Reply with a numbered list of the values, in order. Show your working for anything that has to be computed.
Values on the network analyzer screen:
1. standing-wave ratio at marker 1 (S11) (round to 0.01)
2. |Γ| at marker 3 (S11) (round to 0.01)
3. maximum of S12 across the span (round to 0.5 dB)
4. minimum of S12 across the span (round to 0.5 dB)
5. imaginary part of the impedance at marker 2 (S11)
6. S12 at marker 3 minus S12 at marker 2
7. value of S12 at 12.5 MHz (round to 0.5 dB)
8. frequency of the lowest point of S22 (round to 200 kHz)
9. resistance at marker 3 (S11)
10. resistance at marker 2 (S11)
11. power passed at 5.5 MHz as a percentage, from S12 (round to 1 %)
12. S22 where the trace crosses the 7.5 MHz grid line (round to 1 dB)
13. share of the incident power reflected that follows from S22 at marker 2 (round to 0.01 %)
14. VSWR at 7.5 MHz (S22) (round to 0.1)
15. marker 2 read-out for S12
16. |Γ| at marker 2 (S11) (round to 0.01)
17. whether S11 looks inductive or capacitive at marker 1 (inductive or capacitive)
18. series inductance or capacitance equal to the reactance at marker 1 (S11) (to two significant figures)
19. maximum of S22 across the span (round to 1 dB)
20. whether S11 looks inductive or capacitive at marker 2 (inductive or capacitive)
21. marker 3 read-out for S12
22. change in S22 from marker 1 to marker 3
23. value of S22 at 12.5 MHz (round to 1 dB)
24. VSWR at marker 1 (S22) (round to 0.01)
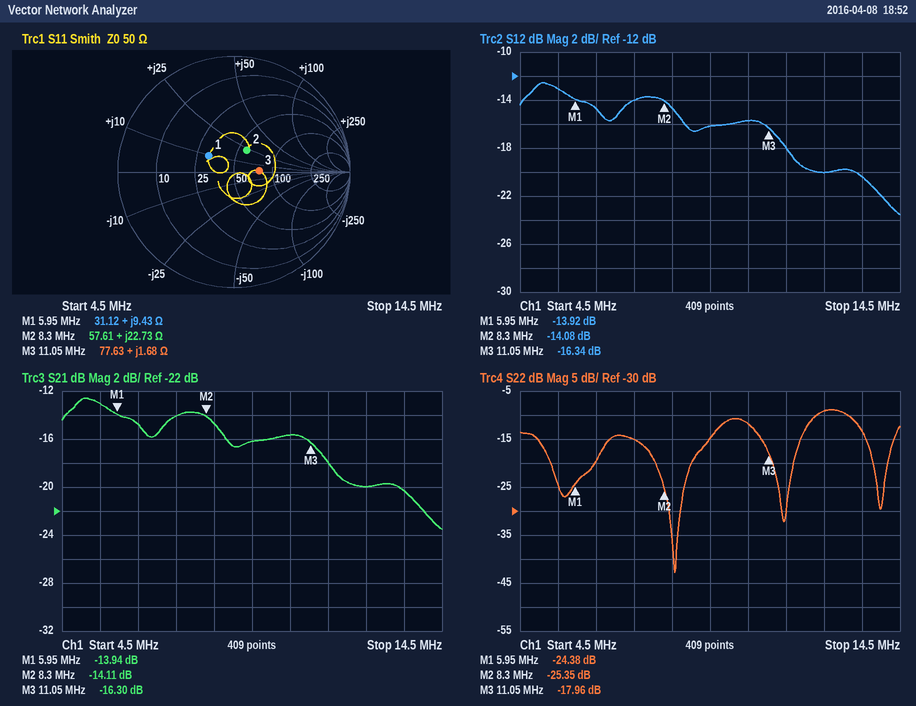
1. 1.70
2. 0.22
3. -12.5 dB
4. -23.5 dB
5. +22.73 Ω
6. -16.34 − (-14.08) = -2.26 dB
7. -20.0 dB
8. 8.6 MHz
9. 77.63 Ω
10. 57.61 Ω
11. 10^(-13/10) ≈ 5 %
12. -15 dB
13. 10^(-25.35/10) ≈ 0.29 %
14. |Γ| = 10^(-15/20) = 0.1778; VSWR = (1 + 0.1778)/(1 − 0.1778) ≈ 1.4
15. -14.08 dB
16. 0.22
17. inductive
18. L = 9.43 Ω/(2π × 5.95 MHz) ≈ 252 nH, so 250 nH to two significant figures
19. -9 dB
20. inductive
21. -16.34 dB
22. -17.96 − (-24.38) = 6.42 dB
23. -9 dB
24. (1 + 0.0604)/(1 − 0.0604) ≈ 1.13
